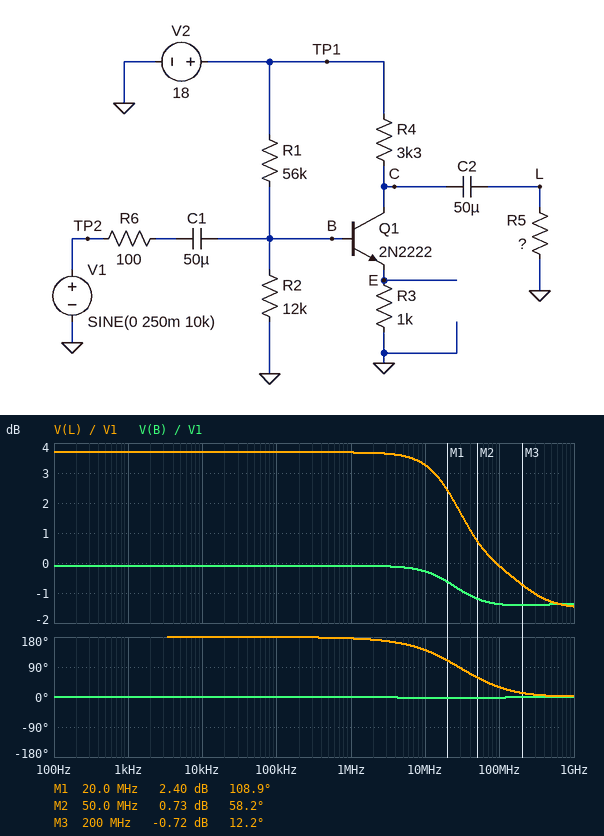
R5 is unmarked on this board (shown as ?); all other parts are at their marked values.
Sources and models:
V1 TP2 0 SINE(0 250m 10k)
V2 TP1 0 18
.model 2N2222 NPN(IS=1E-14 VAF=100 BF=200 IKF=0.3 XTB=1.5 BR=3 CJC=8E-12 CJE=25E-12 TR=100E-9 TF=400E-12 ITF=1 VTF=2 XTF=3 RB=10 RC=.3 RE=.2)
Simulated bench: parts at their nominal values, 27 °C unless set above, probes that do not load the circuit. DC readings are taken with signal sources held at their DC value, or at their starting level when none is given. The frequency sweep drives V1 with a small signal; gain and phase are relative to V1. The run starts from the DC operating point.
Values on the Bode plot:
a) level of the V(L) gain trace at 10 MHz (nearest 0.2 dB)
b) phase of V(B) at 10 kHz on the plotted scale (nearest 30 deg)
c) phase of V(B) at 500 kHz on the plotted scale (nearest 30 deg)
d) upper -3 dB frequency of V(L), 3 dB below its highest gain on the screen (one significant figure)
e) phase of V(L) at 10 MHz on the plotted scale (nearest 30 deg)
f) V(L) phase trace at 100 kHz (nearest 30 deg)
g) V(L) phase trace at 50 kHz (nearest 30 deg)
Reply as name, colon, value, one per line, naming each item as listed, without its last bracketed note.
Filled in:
level of the V(L) gain trace at 10 MHz: 3.2 dB
phase of V(B) at 10 kHz on the plotted scale: 0 deg
phase of V(B) at 500 kHz on the plotted scale: 0 deg
upper -3 dB frequency of V(L), 3 dB below its highest gain on the screen: 50 MHz
phase of V(L) at 10 MHz on the plotted scale: 150 deg
V(L) phase trace at 100 kHz: 180 deg
V(L) phase trace at 50 kHz: 180 deg
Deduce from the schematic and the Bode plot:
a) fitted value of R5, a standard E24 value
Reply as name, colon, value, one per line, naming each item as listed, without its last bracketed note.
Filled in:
fitted value of R5, a standard E24 value: 3 kΩ
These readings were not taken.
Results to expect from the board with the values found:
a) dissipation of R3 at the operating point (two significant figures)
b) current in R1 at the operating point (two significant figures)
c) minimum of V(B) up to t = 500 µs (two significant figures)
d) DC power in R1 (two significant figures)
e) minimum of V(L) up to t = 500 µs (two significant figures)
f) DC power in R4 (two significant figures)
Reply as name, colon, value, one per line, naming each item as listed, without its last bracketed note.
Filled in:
dissipation of R3 at the operating point: 5.7 mW
current in R1 at the operating point: 270 µA
minimum of V(B) up to t = 500 µs: 2.8 V
DC power in R1: 4.0 mW
minimum of V(L) up to t = 500 µs: -380 mV
DC power in R4: 19 mW
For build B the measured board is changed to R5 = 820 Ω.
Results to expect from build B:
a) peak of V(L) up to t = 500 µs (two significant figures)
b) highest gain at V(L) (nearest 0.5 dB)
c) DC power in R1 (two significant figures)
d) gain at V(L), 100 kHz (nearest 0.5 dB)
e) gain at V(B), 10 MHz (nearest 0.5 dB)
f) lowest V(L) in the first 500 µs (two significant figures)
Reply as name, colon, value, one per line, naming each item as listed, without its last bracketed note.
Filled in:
peak of V(L) up to t = 500 µs: 160 mV
highest gain at V(L): -1.5 dB
DC power in R1: 4.0 mW
gain at V(L), 100 kHz: -4.0 dB
gain at V(B), 10 MHz: 0 dB
lowest V(L) in the first 500 µs: -160 mV
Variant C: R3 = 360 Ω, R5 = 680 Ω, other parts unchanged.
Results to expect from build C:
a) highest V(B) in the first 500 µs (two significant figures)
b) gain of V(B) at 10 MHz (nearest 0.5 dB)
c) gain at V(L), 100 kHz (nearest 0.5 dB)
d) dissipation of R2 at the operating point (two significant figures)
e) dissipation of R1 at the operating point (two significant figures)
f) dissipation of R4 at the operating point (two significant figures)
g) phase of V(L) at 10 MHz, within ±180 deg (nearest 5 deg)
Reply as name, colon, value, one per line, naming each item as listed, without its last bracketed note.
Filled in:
highest V(B) in the first 500 µs: 2.7 V
gain of V(B) at 10 MHz: -3.0 dB
gain at V(L), 100 kHz: -13.5 dB
dissipation of R2 at the operating point: 510 µW
dissipation of R1 at the operating point: 4.3 mW
dissipation of R4 at the operating point: 79 mW
phase of V(L) at 10 MHz, within ±180 deg: 5 deg
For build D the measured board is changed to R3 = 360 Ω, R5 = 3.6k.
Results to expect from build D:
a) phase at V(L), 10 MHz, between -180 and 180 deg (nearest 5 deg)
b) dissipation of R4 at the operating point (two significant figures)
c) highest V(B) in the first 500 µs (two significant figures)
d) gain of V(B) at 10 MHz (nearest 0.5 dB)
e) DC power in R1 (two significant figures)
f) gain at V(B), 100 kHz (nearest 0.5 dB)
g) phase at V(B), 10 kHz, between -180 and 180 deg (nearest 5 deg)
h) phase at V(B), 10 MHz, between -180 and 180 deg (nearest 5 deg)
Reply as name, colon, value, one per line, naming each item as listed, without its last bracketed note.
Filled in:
phase at V(L), 10 MHz, between -180 and 180 deg: 5 deg
dissipation of R4 at the operating point: 79 mW
highest V(B) in the first 500 µs: 2.7 V
gain of V(B) at 10 MHz: -2.5 dB
DC power in R1: 4.3 mW
gain at V(B), 100 kHz: -2.0 dB
phase at V(B), 10 kHz, between -180 and 180 deg: 0 deg
phase at V(B), 10 MHz, between -180 and 180 deg: 0 deg
